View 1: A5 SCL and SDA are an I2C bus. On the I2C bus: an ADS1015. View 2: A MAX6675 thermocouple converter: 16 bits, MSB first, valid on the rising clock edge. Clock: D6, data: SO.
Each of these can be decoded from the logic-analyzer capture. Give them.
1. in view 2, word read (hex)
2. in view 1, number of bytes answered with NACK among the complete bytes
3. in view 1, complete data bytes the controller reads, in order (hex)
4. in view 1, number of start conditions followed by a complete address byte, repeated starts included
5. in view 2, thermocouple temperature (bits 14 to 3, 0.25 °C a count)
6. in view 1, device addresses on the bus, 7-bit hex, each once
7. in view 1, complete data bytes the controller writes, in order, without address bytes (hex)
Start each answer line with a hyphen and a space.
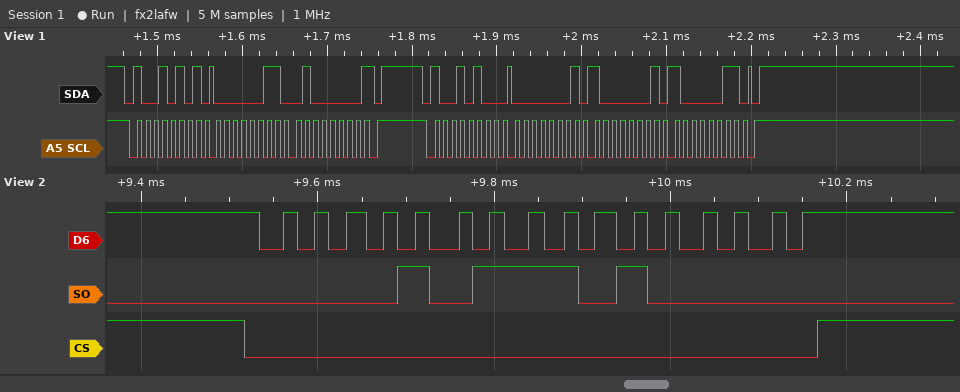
- 0x0BA0
- 1
- 03 40
- 2
- 93.00 °C
- 0x4A
- 01 81 83
